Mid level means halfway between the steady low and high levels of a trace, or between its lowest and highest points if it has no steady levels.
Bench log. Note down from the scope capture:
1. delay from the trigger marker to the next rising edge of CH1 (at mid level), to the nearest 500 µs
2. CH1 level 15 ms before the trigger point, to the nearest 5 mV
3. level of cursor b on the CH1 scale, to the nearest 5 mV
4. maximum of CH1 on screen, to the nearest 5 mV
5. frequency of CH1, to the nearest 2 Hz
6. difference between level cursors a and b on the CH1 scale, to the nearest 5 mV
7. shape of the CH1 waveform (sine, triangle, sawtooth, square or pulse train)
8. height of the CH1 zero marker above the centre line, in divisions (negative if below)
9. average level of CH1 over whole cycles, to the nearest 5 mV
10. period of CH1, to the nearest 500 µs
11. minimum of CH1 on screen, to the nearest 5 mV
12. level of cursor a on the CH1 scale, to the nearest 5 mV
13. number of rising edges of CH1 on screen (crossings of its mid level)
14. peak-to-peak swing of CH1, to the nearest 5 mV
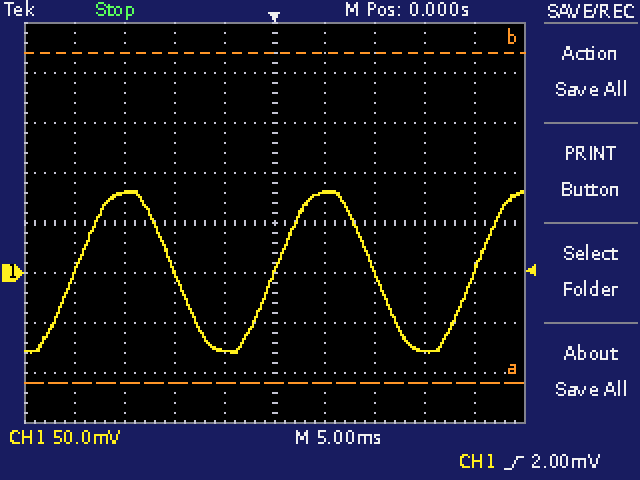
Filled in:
20.0 ms
80 mV
220 mV
80 mV
50 Hz
330 mV
sine
-1.0 div
0 mV
20.0 ms
-80 mV
-110 mV
3
160 mV
